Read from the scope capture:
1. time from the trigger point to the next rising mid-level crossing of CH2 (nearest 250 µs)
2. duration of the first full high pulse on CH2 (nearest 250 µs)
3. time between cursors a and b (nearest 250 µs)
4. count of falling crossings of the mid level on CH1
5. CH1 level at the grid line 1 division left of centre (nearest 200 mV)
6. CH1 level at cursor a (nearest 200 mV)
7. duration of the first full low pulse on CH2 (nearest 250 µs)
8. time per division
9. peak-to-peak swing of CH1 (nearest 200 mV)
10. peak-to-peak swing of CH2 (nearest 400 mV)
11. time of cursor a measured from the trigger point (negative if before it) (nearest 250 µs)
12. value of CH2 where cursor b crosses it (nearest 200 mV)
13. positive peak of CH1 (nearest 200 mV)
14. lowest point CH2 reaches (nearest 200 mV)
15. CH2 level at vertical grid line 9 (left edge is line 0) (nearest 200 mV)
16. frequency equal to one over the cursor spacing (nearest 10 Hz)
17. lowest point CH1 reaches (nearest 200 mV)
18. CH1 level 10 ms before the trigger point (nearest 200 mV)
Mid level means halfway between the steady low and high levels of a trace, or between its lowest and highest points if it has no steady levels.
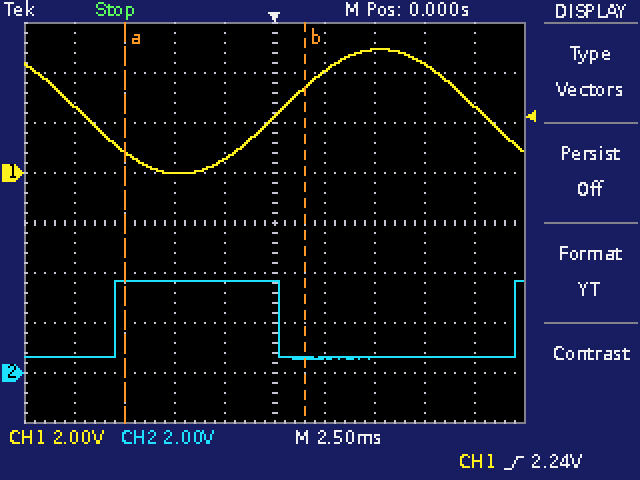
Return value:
12.00 ms
8.25 ms
9.00 ms
2
600 mV
800 mV
11.75 ms
2.5 ms
5.0 V
3.2 V
-7.50 ms
600 mV
5.0 V
600 mV
600 mV
110 Hz
0.0 V
2.6 V
